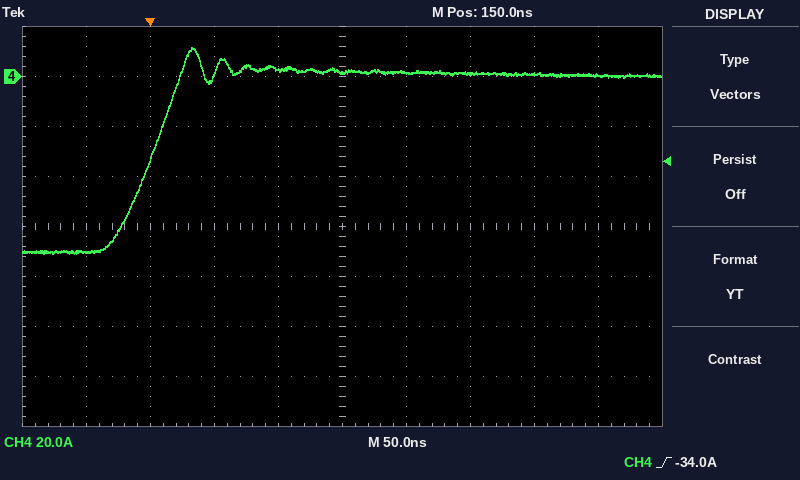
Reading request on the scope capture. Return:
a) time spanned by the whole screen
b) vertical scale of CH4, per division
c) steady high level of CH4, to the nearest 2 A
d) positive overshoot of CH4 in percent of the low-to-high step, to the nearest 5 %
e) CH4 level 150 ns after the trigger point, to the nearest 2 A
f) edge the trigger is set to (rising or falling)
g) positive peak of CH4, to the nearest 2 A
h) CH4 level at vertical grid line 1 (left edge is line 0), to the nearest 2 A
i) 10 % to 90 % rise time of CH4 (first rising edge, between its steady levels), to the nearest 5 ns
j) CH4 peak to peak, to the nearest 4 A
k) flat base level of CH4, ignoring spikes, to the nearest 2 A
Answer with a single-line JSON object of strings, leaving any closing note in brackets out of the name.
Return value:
{"time spanned by the whole screen": "500 ns", "vertical scale of CH4, per division": "20 A", "steady high level of CH4, to the nearest 2 A": "2 A", "positive overshoot of CH4 in percent of the low-to-high step, to the nearest 5 %": "15 %", "CH4 level 150 ns after the trigger point, to the nearest 2 A": "2 A", "edge the trigger is set to": "rising", "positive peak of CH4, to the nearest 2 A": "12 A", "CH4 level at vertical grid line 1 (left edge is line 0), to the nearest 2 A": "-70 A", "10 % to 90 % rise time of CH4 (first rising edge, between its steady levels), to the nearest 5 ns": "45 ns", "CH4 peak to peak, to the nearest 4 A": "84 A", "flat base level of CH4, ignoring spikes, to the nearest 2 A": "-70 A"}
